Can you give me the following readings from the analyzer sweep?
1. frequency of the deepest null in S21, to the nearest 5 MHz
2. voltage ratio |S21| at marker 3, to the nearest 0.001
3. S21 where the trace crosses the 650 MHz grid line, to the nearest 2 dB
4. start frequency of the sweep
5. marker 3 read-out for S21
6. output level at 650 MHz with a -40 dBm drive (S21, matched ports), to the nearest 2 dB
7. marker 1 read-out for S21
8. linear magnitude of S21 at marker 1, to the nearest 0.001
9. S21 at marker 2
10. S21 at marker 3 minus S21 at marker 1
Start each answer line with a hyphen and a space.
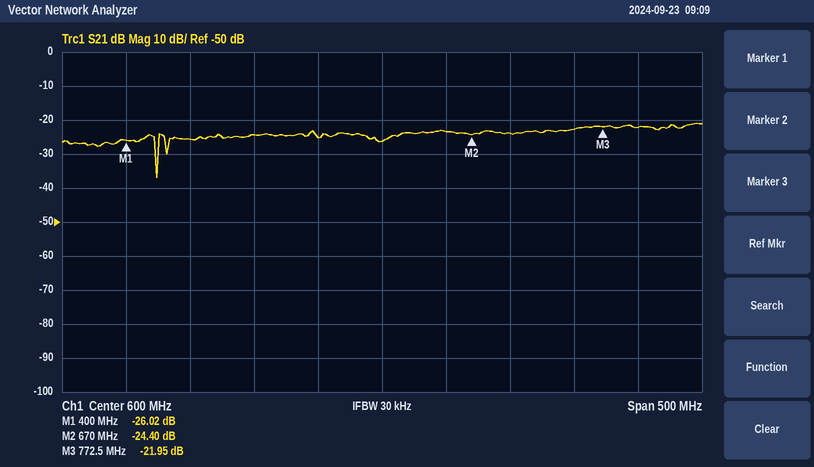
- 425 MHz
- 0.080
- -24 dB
- 350 MHz
- -21.95 dB
- -64 dBm
- -26.02 dB
- 0.050
- -24.40 dB
- 4.07 dB
